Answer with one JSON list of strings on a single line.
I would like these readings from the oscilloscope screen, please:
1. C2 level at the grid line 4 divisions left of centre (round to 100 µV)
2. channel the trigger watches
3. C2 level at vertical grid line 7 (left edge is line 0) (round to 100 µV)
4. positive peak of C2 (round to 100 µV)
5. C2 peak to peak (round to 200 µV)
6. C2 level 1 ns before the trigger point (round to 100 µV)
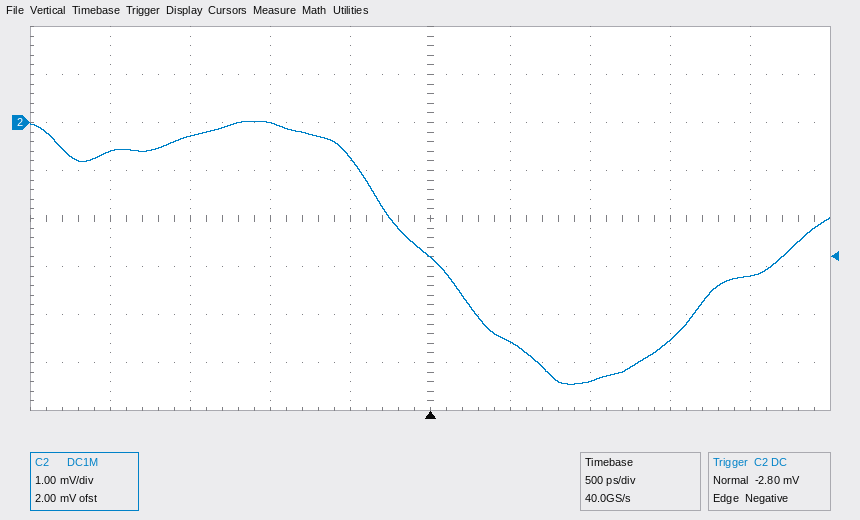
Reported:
["-600 µV", "C2", "-5.4 mV", "0.0 mV", "5.4 mV", "0.0 mV"]
